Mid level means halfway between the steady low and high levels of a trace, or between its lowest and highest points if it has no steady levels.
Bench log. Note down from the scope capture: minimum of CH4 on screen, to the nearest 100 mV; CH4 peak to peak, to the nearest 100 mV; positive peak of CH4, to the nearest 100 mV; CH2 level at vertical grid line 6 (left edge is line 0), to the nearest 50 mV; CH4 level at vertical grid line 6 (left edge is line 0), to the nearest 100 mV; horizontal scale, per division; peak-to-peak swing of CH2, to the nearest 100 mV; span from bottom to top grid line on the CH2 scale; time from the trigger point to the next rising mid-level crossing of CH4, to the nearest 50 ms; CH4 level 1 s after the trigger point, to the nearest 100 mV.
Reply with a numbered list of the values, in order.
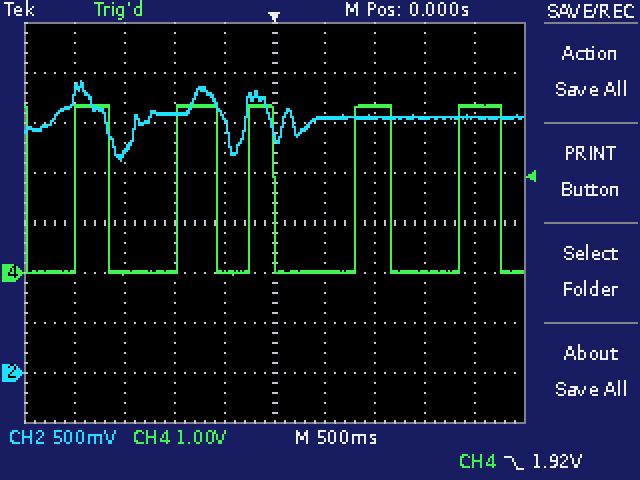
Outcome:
1. 0.0 V
2. 3.4 V
3. 3.4 V
4. 2.55 V
5. 0.0 V
6. 500 ms
7. 800 mV
8. 4 V
9. 800 ms
10. 3.3 V
